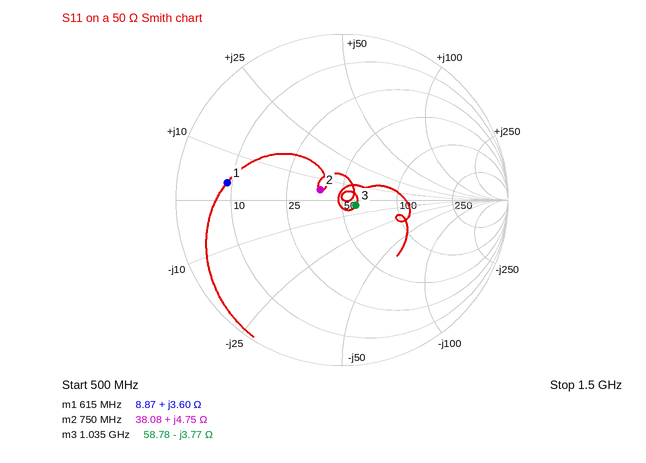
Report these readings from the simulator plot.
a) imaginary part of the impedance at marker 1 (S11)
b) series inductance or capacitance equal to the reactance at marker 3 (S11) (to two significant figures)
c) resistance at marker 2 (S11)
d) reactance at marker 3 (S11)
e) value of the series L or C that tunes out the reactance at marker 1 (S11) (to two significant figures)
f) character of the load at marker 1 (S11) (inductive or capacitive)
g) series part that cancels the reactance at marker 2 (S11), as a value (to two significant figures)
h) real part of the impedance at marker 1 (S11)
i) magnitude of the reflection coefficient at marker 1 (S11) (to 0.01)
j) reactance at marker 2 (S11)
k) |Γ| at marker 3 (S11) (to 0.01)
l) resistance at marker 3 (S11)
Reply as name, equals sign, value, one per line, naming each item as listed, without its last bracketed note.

imaginary part of the impedance at marker 1 = +3.60 Ω
series inductance or capacitance equal to the reactance at marker 3 (S11) = 41 pF
resistance at marker 2 = 38.08 Ω
reactance at marker 3 = -3.77 Ω
value of the series L or C that tunes out the reactance at marker 1 (S11) = 72 pF
character of the load at marker 1 (S11) = inductive
series part that cancels the reactance at marker 2 (S11), as a value = 45 pF
real part of the impedance at marker 1 = 8.87 Ω
magnitude of the reflection coefficient at marker 1 (S11) = 0.70
reactance at marker 2 = +4.75 Ω
|Γ| at marker 3 (S11) = 0.09
resistance at marker 3 = 58.78 Ω
